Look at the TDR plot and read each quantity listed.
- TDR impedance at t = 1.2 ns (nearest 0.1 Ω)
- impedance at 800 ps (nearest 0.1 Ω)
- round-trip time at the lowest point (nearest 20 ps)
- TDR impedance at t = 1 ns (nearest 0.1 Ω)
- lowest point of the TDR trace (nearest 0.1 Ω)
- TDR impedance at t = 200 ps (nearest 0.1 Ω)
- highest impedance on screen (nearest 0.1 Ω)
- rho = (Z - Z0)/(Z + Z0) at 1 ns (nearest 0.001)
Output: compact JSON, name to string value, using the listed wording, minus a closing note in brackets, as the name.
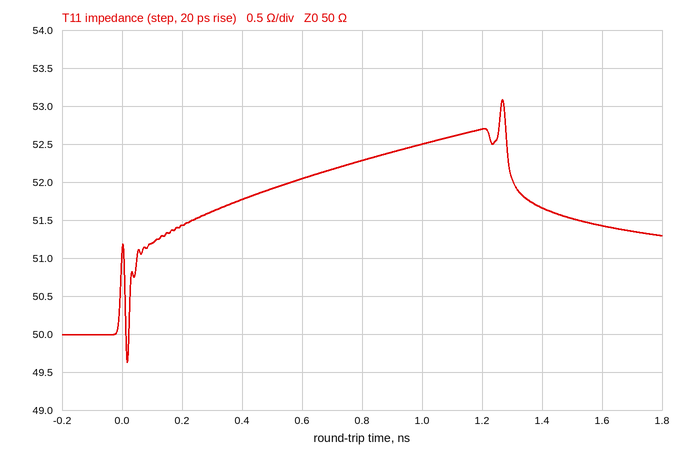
{"TDR impedance at t = 1.2 ns": "52.7 Ω", "impedance at 800 ps": "52.3 Ω", "round-trip time at the lowest point": "20 ps", "TDR impedance at t = 1 ns": "52.5 Ω", "lowest point of the TDR trace": "49.6 Ω", "TDR impedance at t = 200 ps": "51.4 Ω", "highest impedance on screen": "53.1 Ω", "rho = (Z - Z0)/(Z + Z0) at 1 ns": "+0.024"}
